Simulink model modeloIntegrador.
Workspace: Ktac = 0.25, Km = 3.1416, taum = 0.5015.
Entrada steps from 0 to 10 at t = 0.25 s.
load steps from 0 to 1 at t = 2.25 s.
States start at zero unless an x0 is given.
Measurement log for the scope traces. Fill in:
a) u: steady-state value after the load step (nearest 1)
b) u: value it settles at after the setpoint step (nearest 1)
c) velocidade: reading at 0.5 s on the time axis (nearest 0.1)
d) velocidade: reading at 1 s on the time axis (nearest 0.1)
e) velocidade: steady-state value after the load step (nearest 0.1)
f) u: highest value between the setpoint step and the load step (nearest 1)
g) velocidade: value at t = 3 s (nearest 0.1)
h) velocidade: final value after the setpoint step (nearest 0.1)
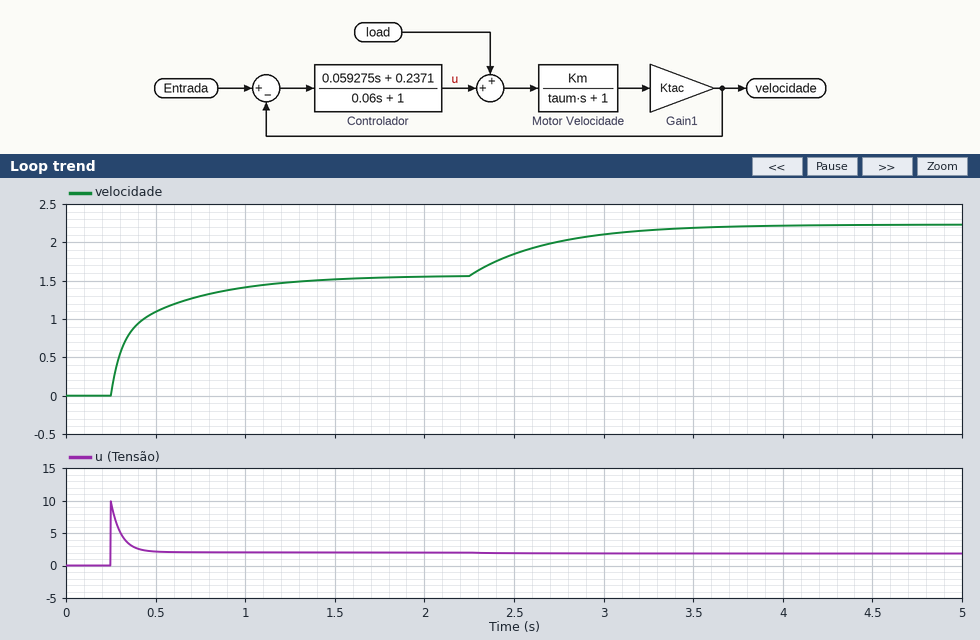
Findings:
2
2
1.1
1.4
2.2
10
2.1
1.6
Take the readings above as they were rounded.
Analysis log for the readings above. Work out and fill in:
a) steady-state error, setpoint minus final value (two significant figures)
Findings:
8.4
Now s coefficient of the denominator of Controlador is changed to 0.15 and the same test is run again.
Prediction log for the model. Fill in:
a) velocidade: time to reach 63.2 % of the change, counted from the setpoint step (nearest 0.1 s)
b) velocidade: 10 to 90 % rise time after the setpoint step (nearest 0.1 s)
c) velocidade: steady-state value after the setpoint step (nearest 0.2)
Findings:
0.3 s
0.8 s
1.6
